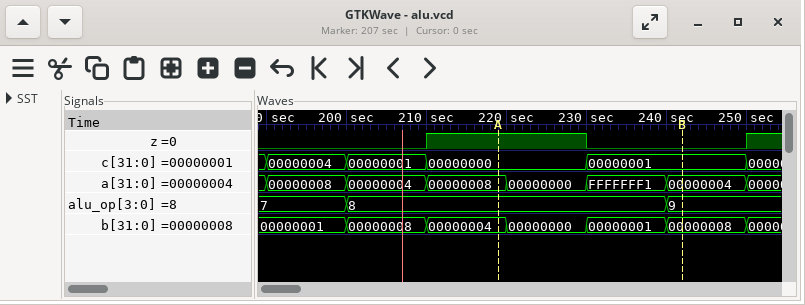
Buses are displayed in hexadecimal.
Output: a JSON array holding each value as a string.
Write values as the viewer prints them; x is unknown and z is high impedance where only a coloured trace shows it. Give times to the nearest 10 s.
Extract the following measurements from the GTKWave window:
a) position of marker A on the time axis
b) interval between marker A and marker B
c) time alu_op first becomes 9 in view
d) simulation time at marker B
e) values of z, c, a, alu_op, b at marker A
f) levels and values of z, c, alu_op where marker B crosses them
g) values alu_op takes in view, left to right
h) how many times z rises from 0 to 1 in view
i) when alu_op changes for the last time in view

["220 s", "20 s", "240 s", "240 s", "z=1, c=00000000, a=00000008, alu_op=8, b=00000004", "z=0, c=00000001, alu_op=9", "7, 8, 9", "2", "240 s"]
